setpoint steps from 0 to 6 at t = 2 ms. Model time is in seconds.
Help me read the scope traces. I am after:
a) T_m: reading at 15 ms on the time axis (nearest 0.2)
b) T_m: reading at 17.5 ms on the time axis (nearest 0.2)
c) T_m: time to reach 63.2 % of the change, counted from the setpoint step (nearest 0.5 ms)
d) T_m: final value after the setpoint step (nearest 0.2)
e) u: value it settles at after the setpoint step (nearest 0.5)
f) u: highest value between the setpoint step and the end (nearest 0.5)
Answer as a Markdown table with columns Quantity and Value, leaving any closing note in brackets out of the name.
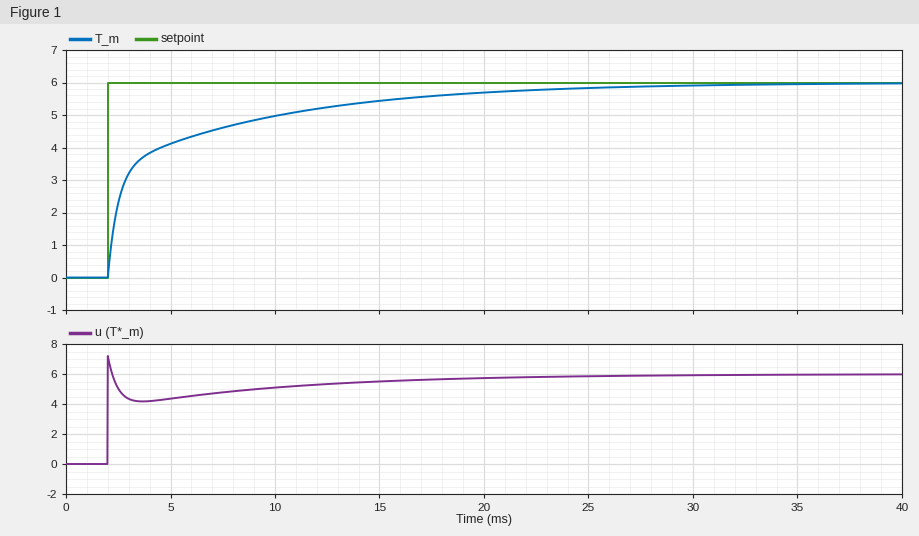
| Quantity | Value |
|---|---|
| T_m: reading at 15 ms on the time axis | 5.4 |
| T_m: reading at 17.5 ms on the time axis | 5.6 |
| T_m: time to reach 63.2 % of the change, counted from the setpoint step | 2.0 ms |
| T_m: final value after the setpoint step | 6.0 |
| u: value it settles at after the setpoint step | 6.0 |
| u: highest value between the setpoint step and the end | 7.0 |
